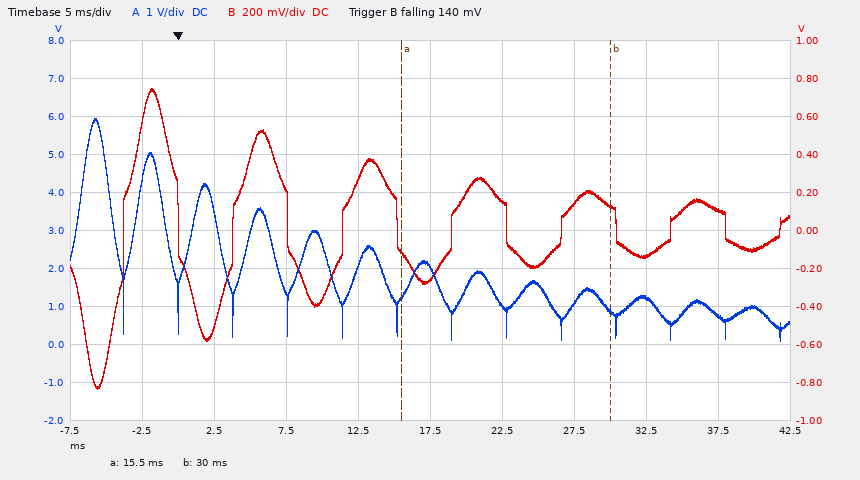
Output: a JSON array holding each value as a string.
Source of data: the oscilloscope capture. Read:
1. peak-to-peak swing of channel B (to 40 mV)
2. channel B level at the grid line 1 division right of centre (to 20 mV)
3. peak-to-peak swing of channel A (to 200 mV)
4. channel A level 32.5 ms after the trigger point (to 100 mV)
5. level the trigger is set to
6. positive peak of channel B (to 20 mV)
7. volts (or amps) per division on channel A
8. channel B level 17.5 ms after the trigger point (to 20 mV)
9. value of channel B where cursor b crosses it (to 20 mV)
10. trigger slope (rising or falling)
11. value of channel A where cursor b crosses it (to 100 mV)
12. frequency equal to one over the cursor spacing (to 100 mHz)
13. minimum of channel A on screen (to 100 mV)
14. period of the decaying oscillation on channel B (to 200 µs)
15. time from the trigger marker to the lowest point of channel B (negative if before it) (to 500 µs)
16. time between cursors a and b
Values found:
["1.56 V", "160 mV", "5.8 V", "1.2 V", "140 mV", "740 mV", "1 V", "-260 mV", "120 mV", "falling", "900 mV", "69.0 Hz", "100 mV", "7.6 ms", "-5.5 ms", "14.5 ms"]
